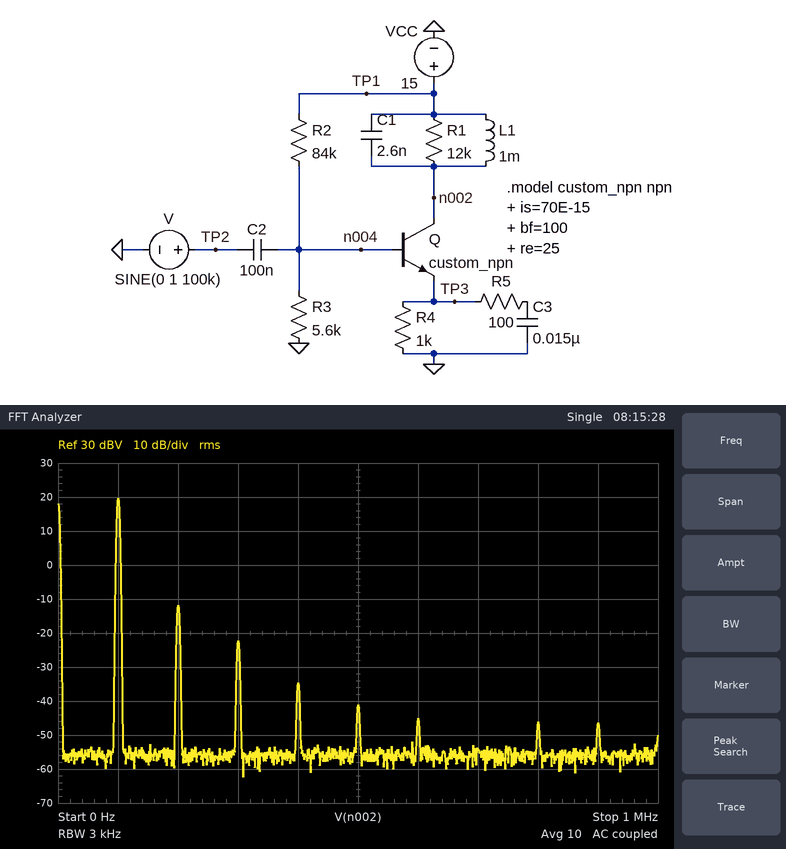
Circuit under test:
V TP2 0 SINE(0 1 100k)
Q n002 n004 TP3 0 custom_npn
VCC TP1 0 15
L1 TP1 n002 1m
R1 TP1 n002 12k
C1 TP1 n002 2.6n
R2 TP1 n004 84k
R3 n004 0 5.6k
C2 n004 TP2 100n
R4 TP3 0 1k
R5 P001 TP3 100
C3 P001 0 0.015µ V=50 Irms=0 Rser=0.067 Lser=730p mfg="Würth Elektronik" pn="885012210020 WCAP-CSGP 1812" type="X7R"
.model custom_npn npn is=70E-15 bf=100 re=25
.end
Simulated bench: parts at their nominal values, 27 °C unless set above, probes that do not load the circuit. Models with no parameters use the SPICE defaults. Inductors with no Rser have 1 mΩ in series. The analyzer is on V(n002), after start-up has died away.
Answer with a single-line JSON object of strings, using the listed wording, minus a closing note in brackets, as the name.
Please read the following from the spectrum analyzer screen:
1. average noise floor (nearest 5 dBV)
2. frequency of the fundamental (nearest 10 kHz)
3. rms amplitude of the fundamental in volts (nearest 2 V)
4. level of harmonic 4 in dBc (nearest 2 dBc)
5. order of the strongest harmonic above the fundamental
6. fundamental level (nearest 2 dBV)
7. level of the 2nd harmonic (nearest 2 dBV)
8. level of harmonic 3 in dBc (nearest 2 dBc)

{"average noise floor": "-55 dBV", "frequency of the fundamental": "100 kHz", "rms amplitude of the fundamental in volts": "10 V", "level of harmonic 4 in dBc": "-54 dBc", "order of the strongest harmonic above the fundamental": "2", "fundamental level": "20 dBV", "level of the 2nd harmonic": "-12 dBV", "level of harmonic 3 in dBc": "-42 dBc"}
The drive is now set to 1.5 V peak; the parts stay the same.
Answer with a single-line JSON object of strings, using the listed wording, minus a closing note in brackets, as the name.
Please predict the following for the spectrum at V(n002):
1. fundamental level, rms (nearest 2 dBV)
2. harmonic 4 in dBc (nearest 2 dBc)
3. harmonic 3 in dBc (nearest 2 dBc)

{"fundamental level, rms": "20 dBV", "harmonic 4 in dBc": "-48 dBc", "harmonic 3 in dBc": "-40 dBc"}
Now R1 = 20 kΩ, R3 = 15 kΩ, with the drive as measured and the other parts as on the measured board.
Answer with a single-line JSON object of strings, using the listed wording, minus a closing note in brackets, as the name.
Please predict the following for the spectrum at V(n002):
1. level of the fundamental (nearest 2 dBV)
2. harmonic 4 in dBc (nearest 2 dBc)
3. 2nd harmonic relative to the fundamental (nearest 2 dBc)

{"level of the fundamental": "20 dBV", "harmonic 4 in dBc": "-48 dBc", "2nd harmonic relative to the fundamental": "-34 dBc"}
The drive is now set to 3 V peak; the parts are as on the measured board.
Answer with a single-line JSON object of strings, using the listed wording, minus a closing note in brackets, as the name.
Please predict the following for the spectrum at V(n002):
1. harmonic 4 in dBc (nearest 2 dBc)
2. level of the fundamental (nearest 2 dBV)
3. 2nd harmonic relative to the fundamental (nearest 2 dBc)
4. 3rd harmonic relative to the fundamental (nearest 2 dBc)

{"harmonic 4 in dBc": "-44 dBc", "level of the fundamental": "20 dBV", "2nd harmonic relative to the fundamental": "-30 dBc", "3rd harmonic relative to the fundamental": "-38 dBc"}
